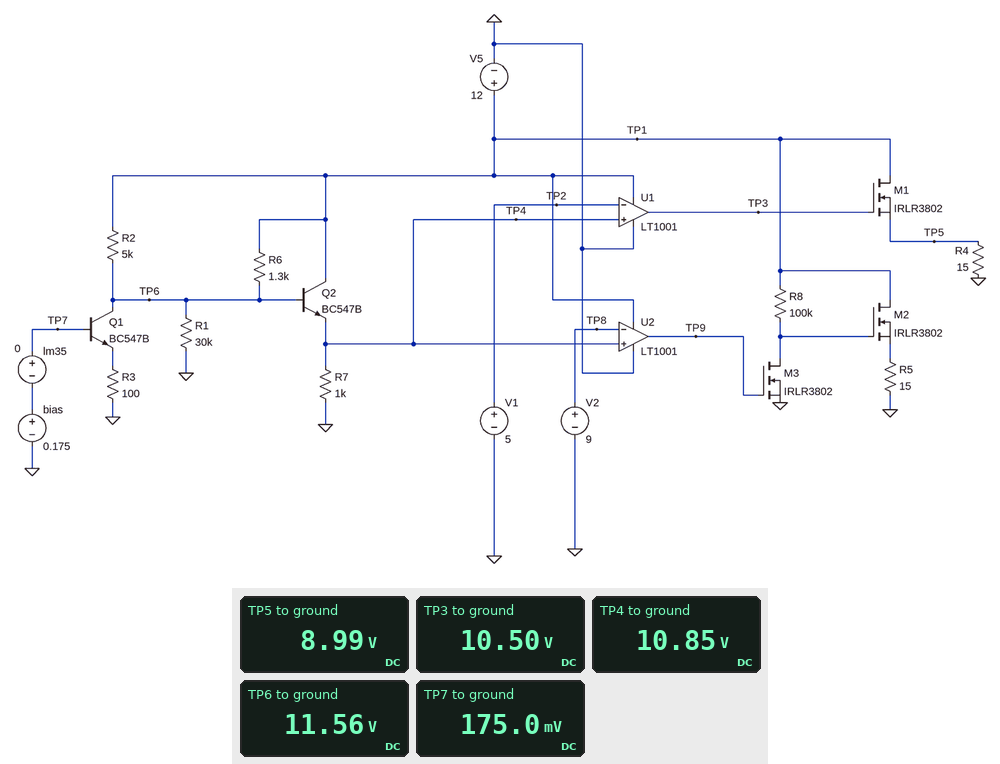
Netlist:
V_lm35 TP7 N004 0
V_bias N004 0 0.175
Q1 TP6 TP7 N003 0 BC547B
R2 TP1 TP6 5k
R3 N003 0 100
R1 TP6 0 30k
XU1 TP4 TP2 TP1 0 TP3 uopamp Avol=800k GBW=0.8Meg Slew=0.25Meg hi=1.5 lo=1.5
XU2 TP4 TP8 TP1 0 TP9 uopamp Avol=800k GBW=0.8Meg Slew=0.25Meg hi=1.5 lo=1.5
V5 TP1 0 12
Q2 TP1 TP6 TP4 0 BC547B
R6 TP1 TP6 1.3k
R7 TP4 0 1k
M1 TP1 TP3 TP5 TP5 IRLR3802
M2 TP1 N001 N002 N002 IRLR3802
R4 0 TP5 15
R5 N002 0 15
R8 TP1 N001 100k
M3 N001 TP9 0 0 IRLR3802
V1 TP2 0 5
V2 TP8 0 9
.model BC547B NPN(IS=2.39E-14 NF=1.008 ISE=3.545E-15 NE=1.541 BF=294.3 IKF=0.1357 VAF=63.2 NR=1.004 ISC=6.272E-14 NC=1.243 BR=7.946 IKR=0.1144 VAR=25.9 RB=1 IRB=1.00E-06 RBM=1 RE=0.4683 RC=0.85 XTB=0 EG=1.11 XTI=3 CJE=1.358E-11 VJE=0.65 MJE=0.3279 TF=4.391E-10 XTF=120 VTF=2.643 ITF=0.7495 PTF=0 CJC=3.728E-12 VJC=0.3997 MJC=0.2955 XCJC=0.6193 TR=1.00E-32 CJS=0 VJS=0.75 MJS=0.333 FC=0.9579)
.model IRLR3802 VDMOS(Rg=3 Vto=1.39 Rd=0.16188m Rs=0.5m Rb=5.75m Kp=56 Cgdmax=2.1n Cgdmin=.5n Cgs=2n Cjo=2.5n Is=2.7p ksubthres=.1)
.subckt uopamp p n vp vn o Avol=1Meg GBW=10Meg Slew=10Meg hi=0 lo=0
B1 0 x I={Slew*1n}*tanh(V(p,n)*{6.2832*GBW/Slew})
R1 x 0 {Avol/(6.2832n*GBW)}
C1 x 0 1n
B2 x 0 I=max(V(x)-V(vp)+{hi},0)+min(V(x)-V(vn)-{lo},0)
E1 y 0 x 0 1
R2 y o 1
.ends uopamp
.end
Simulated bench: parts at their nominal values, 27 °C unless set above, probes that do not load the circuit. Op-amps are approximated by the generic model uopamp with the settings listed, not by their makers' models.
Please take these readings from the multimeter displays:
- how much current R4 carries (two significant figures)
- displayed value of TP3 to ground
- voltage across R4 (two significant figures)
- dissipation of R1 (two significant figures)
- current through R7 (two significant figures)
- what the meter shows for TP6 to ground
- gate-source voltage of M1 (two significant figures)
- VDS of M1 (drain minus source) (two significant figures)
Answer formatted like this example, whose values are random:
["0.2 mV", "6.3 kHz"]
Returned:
["600 mA", "10.50 V", "9.0 V", "4.5 mW", "11 mA", "11.56 V", "1.5 V", "3.0 V"]
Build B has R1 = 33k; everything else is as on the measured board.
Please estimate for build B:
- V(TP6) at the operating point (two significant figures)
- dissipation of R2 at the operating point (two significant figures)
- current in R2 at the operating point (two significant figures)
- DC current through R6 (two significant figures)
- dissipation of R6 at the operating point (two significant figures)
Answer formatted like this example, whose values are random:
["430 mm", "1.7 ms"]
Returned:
["12 V", "33 µW", "81 µA", "310 µA", "130 µW"]
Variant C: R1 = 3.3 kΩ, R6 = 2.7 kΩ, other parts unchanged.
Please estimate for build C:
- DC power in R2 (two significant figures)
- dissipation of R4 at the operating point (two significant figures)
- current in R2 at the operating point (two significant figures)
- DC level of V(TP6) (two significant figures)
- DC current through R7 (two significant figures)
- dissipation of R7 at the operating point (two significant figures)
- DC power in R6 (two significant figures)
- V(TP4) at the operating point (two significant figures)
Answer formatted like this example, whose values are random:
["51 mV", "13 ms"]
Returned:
["3.5 mW", "5.4 W", "840 µA", "7.8 V", "7.1 mA", "51 mW", "6.5 mW", "7.1 V"]
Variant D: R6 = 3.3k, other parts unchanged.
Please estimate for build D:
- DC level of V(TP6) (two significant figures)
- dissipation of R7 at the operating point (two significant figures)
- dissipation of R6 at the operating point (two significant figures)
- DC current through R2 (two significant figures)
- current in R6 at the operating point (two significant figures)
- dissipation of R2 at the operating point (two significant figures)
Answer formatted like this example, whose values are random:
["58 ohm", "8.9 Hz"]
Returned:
["11 V", "110 mW", "200 µW", "160 µA", "250 µA", "130 µW"]
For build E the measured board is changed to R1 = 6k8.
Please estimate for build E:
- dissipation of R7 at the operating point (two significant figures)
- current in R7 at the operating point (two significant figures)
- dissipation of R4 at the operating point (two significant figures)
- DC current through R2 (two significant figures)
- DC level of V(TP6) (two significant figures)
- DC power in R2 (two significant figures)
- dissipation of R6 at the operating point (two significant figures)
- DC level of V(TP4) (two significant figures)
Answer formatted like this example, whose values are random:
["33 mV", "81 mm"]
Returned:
["94 mW", "9.7 mA", "5.4 W", "320 µA", "10 V", "520 µW", "2.0 mW", "9.7 V"]
